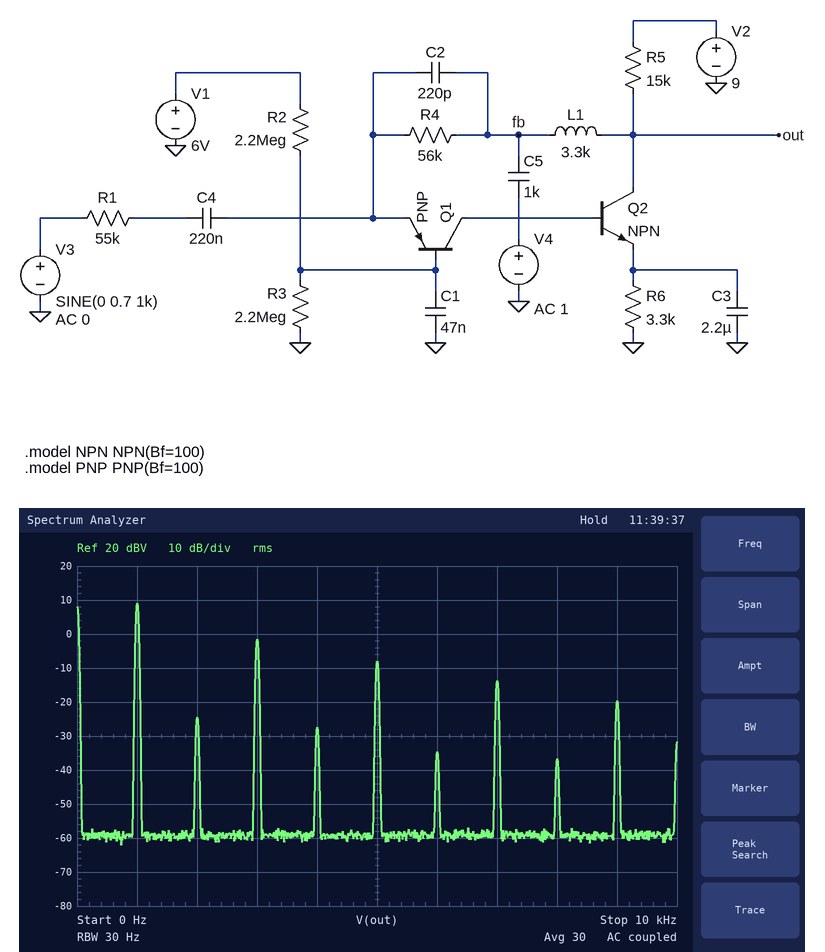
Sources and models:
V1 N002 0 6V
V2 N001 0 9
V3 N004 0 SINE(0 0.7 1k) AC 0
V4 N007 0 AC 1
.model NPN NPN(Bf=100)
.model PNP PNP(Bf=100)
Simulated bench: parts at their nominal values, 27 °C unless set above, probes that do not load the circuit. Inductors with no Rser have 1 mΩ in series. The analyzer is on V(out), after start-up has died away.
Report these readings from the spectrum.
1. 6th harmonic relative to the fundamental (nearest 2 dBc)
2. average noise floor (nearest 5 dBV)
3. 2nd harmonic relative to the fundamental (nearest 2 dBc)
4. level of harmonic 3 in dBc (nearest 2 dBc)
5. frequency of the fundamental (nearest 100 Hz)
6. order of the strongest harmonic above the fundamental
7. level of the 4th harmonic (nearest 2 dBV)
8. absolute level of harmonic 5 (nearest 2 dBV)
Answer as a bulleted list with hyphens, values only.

- -44 dBc
- -60 dBV
- -34 dBc
- -10 dBc
- 1.0 kHz
- 3
- -28 dBV
- -8 dBV
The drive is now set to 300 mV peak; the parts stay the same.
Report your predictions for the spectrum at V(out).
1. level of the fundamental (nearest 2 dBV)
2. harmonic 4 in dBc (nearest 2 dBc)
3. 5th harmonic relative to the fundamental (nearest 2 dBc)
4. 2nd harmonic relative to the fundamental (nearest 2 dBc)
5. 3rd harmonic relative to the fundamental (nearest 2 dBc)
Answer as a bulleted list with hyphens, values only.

- 8 dBV
- -32 dBc
- -28 dBc
- -16 dBc
- -16 dBc
